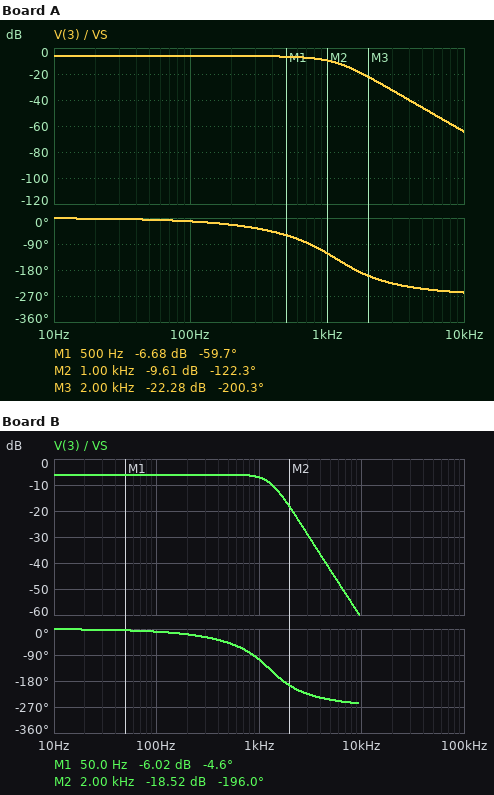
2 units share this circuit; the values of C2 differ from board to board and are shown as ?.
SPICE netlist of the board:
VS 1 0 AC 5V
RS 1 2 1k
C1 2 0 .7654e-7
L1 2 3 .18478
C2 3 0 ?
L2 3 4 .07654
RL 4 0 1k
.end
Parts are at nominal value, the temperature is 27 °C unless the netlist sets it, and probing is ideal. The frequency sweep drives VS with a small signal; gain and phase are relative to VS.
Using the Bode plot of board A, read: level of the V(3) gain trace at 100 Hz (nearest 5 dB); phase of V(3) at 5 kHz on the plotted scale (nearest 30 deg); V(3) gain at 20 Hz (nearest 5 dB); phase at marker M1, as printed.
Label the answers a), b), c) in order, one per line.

a) -5 dB
b) -240 deg
c) -5 dB
d) -59.7 deg
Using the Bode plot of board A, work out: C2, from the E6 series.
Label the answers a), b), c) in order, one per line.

a) 470 nF
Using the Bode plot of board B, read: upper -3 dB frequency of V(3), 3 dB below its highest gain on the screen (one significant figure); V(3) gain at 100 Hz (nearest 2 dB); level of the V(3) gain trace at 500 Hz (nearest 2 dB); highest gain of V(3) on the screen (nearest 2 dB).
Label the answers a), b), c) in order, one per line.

a) 1 kHz
b) -6 dB
c) -6 dB
d) -6 dB
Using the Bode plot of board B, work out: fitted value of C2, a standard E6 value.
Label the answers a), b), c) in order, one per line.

a) 330 nF
